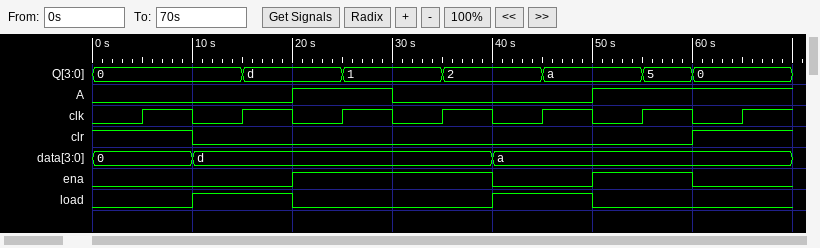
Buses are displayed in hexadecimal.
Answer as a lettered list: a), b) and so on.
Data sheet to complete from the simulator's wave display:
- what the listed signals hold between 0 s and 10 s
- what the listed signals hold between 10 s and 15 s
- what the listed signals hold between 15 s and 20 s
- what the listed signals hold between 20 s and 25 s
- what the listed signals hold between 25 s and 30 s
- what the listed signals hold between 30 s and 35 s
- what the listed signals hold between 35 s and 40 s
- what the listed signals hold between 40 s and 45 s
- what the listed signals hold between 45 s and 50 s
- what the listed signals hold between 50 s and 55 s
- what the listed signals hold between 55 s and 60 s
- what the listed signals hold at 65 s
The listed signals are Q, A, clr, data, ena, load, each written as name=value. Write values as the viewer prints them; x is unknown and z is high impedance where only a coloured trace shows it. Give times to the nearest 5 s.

a) Q=0, A=0, clr=1, data=0, ena=0, load=0
b) Q=0, A=0, clr=0, data=d, ena=0, load=1
c) Q=d, A=0, clr=0, data=d, ena=0, load=1
d) Q=d, A=1, clr=0, data=d, ena=1, load=0
e) Q=1, A=1, clr=0, data=d, ena=1, load=0
f) Q=1, A=0, clr=0, data=d, ena=1, load=0
g) Q=2, A=0, clr=0, data=d, ena=1, load=0
h) Q=2, A=0, clr=0, data=a, ena=0, load=1
i) Q=a, A=0, clr=0, data=a, ena=0, load=1
j) Q=a, A=1, clr=0, data=a, ena=1, load=0
k) Q=5, A=1, clr=0, data=a, ena=1, load=0
l) Q=0, A=1, clr=1, data=a, ena=0, load=0
